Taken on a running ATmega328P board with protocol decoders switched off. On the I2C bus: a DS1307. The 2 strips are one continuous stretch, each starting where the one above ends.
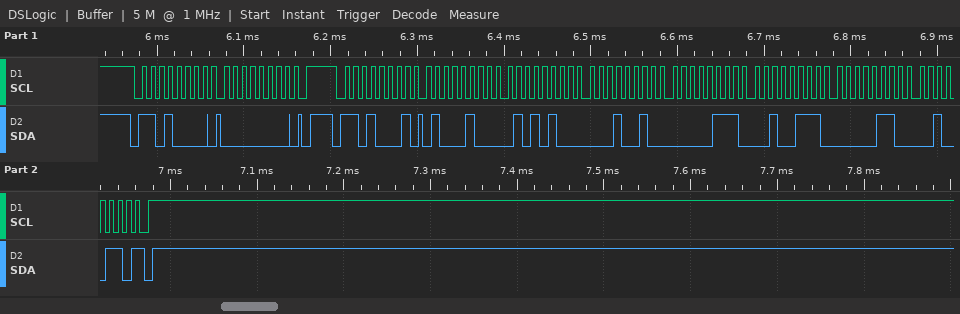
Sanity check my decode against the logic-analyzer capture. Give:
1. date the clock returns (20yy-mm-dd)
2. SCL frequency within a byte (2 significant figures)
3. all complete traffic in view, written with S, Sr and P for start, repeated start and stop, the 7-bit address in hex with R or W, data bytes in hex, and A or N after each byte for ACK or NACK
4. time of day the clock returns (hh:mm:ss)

2026-06-27
100 kHz
S 68W A 00 A P S 68R A 44 A 54 A 12 A 07 A 27 A 06 A 26 N P
12:54:44
